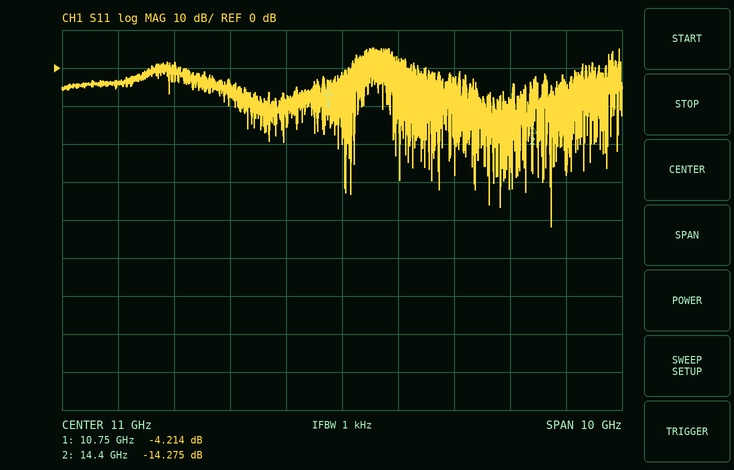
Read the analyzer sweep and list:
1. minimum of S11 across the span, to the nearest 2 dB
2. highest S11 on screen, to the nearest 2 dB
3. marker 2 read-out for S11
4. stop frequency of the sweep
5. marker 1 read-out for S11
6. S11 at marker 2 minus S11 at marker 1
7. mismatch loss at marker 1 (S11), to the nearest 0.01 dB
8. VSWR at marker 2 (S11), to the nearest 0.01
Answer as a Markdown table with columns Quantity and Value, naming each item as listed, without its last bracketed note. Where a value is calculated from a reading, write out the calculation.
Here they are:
| Quantity | Value |
|---|---|
| minimum of S11 across the span, to the nearest 2 dB | -42 dB |
| highest S11 on screen, to the nearest 2 dB | 6 dB |
| marker 2 read-out for S11 | -14.275 dB |
| stop frequency of the sweep | 16 GHz |
| marker 1 read-out for S11 | -4.214 dB |
| S11 at marker 2 minus S11 at marker 1 | -14.275 − (-4.214) = -10.061 dB |
| mismatch loss at marker 1 (S11), to the nearest 0.01 dB | −10 log10(1 − 10^(-4.214/10)) ≈ 2.07 dB |
| VSWR at marker 2 (S11), to the nearest 0.01 | (1 + 0.1933)/(1 − 0.1933) ≈ 1.48 |
